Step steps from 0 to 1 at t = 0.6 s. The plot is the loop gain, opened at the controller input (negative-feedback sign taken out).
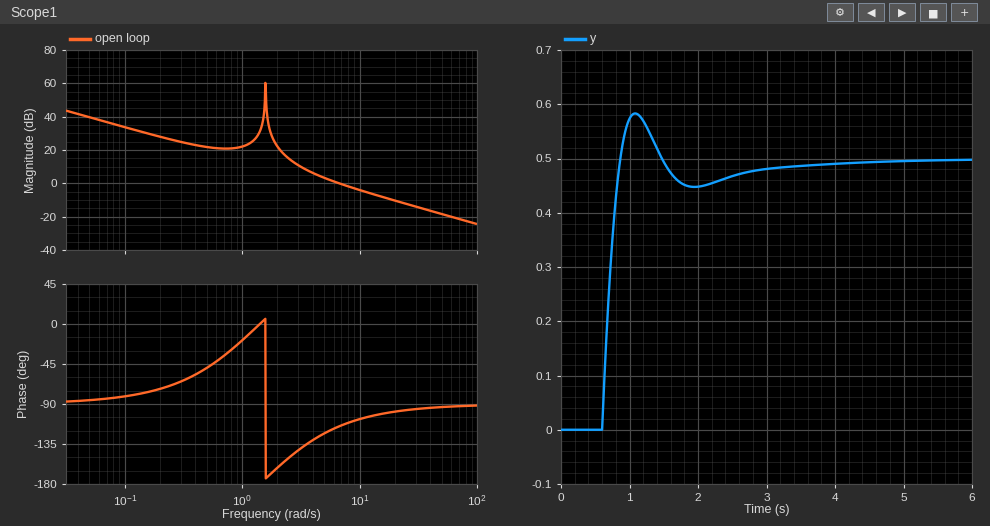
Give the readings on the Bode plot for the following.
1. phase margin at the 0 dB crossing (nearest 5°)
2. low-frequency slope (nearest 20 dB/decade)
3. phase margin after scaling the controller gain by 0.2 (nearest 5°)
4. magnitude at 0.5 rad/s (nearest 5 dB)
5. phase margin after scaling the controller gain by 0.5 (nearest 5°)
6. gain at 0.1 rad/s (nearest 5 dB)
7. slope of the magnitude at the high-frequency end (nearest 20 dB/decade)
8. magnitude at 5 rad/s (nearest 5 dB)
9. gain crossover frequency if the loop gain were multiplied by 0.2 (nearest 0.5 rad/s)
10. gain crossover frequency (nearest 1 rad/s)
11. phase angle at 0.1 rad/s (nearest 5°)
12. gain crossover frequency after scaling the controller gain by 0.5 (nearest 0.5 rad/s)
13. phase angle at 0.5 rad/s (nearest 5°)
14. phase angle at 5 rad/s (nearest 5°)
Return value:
65°
-20 dB/decade
30°
20 dB
50°
35 dB
-20 dB/decade
5 dB
2.5 rad/s
7 rad/s
-80°
4.0 rad/s
-50°
-125°
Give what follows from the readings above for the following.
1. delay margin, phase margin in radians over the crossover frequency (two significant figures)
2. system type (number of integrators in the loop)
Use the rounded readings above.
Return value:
0.16 s
1
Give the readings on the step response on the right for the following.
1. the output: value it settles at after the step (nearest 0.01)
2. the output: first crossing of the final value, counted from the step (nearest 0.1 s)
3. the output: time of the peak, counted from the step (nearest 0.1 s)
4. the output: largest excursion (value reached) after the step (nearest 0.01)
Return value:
0.50
0.3 s
0.5 s
0.58
